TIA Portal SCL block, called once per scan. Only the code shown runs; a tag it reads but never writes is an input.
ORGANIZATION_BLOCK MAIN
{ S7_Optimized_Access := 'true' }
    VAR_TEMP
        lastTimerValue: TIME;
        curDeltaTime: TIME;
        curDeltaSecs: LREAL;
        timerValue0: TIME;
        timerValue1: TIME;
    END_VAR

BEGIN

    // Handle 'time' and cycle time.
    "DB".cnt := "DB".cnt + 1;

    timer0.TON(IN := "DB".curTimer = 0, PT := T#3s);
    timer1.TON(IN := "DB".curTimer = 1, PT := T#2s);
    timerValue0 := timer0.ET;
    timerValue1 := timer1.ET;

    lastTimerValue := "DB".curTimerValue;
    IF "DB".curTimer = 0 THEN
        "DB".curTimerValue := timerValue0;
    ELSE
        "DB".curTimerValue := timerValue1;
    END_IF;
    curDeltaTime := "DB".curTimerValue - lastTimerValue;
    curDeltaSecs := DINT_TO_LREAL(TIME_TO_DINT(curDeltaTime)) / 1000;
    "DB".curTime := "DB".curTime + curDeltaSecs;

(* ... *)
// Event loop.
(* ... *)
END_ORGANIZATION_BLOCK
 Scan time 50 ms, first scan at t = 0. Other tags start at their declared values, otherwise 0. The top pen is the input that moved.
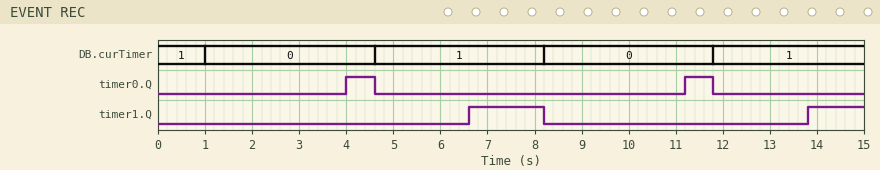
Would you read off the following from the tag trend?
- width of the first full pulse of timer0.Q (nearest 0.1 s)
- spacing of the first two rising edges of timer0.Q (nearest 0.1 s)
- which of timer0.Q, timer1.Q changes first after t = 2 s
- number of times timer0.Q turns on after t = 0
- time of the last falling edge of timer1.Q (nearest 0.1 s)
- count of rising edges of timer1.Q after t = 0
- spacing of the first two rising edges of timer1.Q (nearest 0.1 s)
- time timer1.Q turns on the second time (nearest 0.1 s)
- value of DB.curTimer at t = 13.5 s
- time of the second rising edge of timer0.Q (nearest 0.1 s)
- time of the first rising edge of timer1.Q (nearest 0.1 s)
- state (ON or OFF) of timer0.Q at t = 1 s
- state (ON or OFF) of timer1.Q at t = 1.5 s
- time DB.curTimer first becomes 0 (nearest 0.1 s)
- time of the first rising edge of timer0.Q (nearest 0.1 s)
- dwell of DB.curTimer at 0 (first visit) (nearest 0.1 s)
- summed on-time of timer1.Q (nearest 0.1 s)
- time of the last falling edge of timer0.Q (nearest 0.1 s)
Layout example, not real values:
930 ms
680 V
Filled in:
0.6 s
7.2 s
timer0.Q
2
8.2 s
2
7.2 s
13.8 s
1
11.2 s
6.6 s
OFF
OFF
1.0 s
4.0 s
3.6 s
2.8 s
11.8 s
